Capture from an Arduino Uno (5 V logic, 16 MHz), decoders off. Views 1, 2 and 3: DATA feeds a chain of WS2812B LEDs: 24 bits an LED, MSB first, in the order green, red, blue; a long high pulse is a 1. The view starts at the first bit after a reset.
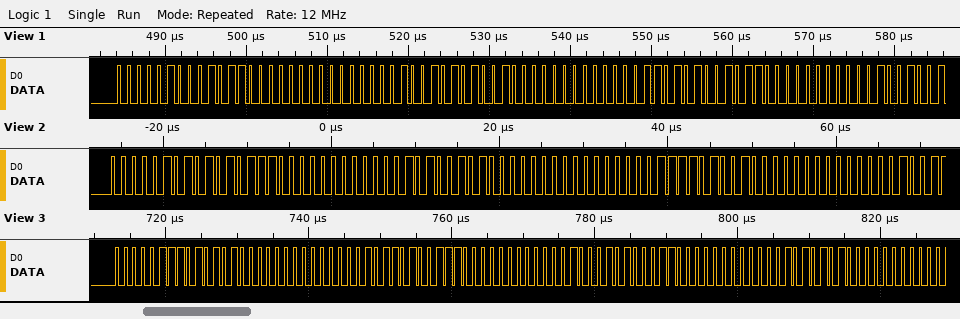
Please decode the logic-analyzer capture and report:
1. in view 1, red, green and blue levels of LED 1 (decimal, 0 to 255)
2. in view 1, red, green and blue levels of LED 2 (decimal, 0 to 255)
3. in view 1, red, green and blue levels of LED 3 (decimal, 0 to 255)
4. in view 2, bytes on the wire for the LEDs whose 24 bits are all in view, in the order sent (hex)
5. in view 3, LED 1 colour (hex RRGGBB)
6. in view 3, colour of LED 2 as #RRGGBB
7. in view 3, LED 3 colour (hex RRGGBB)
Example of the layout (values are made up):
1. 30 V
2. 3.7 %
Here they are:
1. 88, 4, 0
2. 82, 9, 0
3. 75, 13, 0
4. 05 57 00 0A 50 00 0F 48 00
5. #540700
6. #4E0B00
7. #461100
